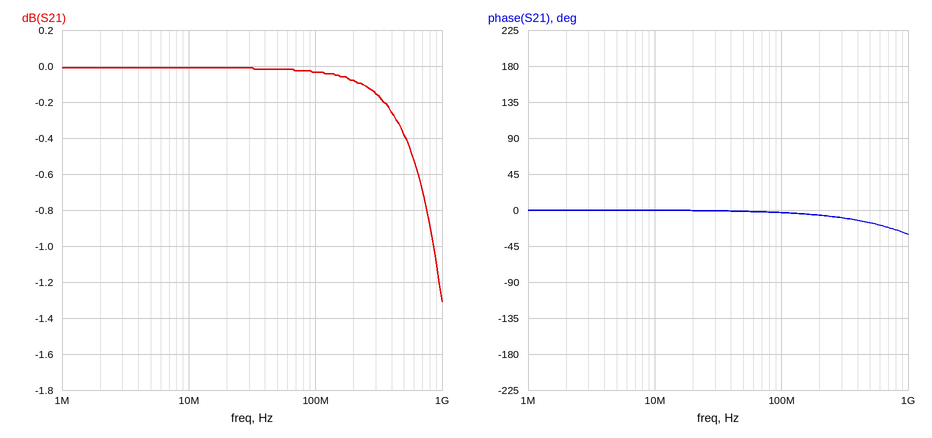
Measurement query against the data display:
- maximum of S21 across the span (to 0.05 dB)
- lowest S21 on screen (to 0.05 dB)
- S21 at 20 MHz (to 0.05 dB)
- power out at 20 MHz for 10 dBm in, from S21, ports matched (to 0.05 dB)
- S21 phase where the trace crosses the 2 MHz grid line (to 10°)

0.00 dB
-1.30 dB
0.00 dB
10.00 dBm
0°
